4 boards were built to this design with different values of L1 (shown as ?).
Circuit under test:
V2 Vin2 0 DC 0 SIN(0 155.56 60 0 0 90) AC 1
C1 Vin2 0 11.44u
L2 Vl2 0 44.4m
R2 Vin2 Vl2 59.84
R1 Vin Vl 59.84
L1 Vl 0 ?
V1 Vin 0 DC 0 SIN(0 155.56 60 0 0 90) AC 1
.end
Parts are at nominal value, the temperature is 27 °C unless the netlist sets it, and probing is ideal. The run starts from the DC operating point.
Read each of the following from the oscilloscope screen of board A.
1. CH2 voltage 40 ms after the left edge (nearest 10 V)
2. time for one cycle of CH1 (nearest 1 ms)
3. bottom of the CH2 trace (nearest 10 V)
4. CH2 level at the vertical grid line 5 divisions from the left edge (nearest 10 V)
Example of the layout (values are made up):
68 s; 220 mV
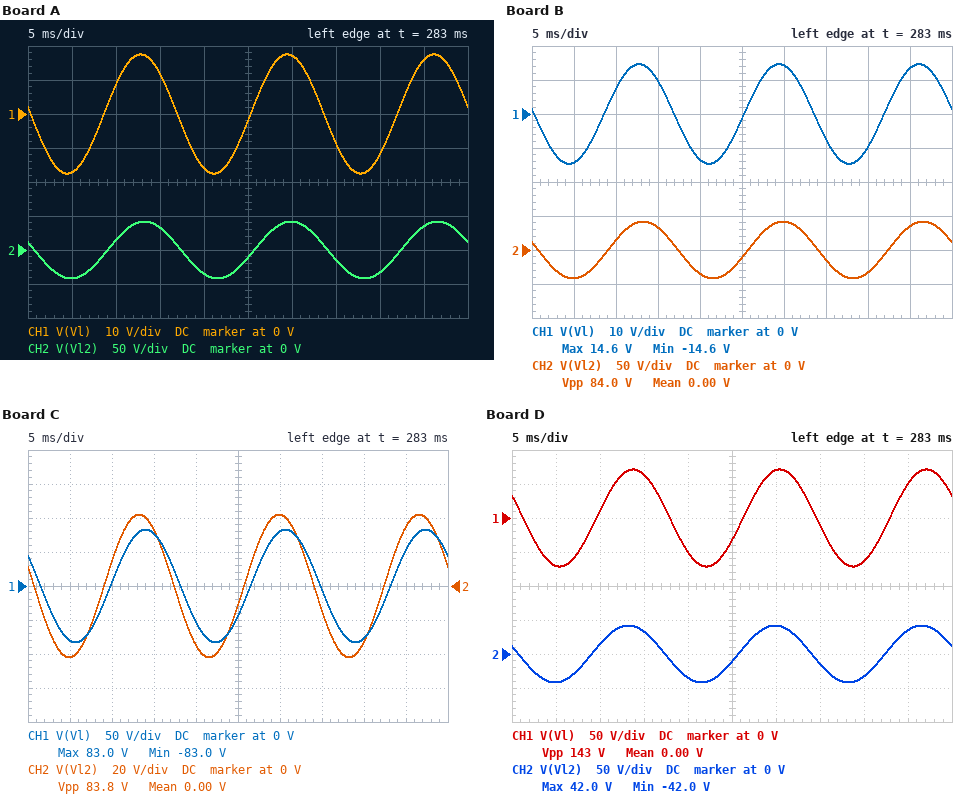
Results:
-30 V; 17 ms; -40 V; -10 V
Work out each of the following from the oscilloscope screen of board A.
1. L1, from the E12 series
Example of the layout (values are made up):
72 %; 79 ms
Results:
18 mH
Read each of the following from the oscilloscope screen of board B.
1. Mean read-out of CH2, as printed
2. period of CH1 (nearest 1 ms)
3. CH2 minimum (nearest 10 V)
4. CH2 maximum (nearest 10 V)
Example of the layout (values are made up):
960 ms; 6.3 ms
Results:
0.00 V; 17 ms; -40 V; 40 V
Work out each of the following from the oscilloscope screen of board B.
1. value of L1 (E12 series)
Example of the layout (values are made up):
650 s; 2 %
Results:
15 mH
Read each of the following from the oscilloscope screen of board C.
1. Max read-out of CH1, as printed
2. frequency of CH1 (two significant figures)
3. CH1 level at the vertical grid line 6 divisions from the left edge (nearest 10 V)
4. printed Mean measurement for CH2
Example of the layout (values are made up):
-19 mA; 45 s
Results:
83.0 V; 60 Hz; 80 V; 0.00 V
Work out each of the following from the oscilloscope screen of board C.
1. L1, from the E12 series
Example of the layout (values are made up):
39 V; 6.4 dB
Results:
100 mH
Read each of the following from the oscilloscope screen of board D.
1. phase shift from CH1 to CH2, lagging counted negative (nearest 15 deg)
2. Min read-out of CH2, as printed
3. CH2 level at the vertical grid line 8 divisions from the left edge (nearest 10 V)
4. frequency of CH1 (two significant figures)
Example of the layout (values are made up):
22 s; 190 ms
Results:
15 deg; -42.0 V; -30 V; 60 Hz
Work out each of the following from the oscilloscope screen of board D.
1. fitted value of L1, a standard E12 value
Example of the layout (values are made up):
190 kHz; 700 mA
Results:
82 mH
